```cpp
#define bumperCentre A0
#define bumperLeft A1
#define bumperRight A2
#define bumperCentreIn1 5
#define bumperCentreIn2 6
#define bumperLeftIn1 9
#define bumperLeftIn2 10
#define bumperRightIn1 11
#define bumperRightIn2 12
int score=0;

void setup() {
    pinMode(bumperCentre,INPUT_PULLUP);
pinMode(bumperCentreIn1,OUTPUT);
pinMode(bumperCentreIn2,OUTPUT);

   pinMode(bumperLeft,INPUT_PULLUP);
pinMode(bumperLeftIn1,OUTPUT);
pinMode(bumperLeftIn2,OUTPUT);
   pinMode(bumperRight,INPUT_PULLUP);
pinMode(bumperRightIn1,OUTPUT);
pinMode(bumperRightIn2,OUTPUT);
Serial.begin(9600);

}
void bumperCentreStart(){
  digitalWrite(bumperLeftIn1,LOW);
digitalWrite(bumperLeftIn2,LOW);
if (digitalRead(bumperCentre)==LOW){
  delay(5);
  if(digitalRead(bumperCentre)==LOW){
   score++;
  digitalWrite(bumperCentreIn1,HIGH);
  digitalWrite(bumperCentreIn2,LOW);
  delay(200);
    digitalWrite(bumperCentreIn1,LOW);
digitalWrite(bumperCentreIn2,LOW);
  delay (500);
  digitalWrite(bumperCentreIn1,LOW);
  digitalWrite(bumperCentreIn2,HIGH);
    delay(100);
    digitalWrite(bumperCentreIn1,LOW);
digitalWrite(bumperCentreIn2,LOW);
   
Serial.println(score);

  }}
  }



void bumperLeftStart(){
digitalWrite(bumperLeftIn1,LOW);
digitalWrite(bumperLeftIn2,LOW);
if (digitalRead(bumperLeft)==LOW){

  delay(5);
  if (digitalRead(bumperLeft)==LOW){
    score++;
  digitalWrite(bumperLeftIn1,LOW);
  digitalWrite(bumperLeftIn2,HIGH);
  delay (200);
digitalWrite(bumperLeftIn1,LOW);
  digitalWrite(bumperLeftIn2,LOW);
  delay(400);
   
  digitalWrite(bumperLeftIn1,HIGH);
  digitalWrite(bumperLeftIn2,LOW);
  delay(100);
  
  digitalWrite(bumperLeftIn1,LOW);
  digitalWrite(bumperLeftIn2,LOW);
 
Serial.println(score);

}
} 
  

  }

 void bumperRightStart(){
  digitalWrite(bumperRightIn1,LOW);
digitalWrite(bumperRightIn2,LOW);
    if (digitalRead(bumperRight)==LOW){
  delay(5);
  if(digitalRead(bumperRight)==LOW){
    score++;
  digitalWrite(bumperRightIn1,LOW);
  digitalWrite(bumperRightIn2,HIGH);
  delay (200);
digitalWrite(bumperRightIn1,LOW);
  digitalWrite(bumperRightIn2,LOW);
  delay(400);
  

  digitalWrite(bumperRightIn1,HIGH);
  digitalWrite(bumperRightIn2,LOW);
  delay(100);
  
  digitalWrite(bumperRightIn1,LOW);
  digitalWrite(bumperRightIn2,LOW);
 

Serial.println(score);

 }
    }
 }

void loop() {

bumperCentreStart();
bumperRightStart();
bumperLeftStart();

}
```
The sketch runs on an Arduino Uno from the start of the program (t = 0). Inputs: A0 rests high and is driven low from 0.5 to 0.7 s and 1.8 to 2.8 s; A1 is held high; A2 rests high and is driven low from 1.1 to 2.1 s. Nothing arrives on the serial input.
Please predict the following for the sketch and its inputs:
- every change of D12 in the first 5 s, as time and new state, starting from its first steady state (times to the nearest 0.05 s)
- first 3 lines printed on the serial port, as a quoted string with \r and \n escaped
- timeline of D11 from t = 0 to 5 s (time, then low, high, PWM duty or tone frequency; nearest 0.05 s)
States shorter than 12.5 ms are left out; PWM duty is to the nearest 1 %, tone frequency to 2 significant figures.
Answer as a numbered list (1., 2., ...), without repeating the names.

1. 0 s low; 1.3 s high; 1.5 s low
2. "1\r\n2\r\n3\r\n"
3. 0 s low; 1.9 s high; 2 s low
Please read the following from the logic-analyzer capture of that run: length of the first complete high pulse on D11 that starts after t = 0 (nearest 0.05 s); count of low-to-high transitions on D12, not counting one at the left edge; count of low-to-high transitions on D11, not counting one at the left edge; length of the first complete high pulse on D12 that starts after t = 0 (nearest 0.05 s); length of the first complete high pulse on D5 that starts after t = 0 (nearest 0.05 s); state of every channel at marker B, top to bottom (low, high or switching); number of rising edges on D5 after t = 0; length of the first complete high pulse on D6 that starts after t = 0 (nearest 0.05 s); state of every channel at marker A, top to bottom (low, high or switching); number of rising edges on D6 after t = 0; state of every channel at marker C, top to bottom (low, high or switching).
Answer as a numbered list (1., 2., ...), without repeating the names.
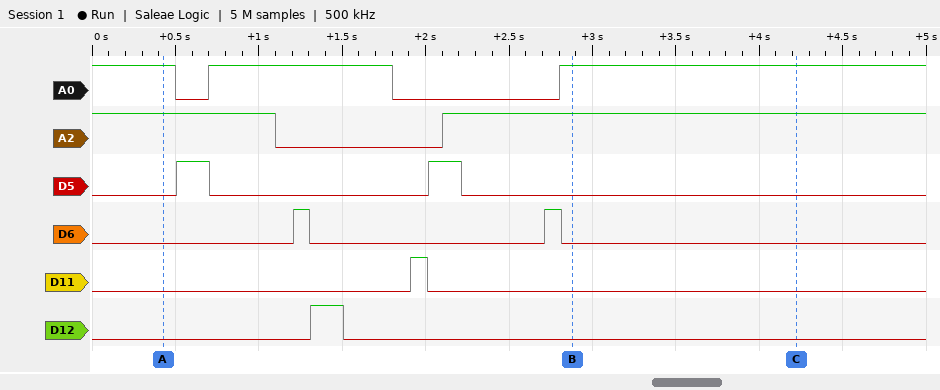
1. 0.10 s
2. 1
3. 1
4. 0.20 s
5. 0.20 s
6. A0 high, A2 high, D5 low, D6 low, D11 low, D12 low
7. 2
8. 0.10 s
9. A0 high, A2 high, D5 low, D6 low, D11 low, D12 low
10. 2
11. A0 high, A2 high, D5 low, D6 low, D11 low, D12 low
